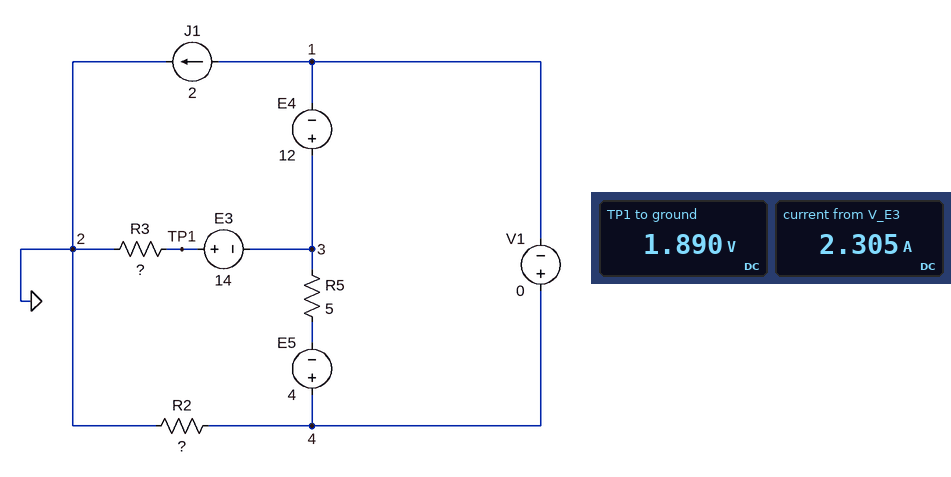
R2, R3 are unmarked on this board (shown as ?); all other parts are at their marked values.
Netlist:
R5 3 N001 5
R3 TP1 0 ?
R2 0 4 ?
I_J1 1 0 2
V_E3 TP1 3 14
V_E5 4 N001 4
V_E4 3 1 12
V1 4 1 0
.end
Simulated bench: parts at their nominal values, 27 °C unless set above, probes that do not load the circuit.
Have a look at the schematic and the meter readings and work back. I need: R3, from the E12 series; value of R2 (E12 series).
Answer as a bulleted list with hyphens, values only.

- 0.82 Ω
- 5.6 Ω
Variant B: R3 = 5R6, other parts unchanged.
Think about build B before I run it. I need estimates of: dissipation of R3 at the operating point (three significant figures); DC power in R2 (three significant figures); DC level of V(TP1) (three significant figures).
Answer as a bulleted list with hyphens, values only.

- 9.78 W
- 61.8 W
- 7.40 V
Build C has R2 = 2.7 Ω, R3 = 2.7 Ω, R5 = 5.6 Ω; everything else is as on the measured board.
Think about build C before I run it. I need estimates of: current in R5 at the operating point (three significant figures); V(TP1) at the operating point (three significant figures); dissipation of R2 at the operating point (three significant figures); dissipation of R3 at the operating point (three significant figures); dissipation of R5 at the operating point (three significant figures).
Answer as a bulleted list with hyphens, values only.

- 2.86 A
- 10.3 V
- 91.3 W
- 39.3 W
- 45.7 W
